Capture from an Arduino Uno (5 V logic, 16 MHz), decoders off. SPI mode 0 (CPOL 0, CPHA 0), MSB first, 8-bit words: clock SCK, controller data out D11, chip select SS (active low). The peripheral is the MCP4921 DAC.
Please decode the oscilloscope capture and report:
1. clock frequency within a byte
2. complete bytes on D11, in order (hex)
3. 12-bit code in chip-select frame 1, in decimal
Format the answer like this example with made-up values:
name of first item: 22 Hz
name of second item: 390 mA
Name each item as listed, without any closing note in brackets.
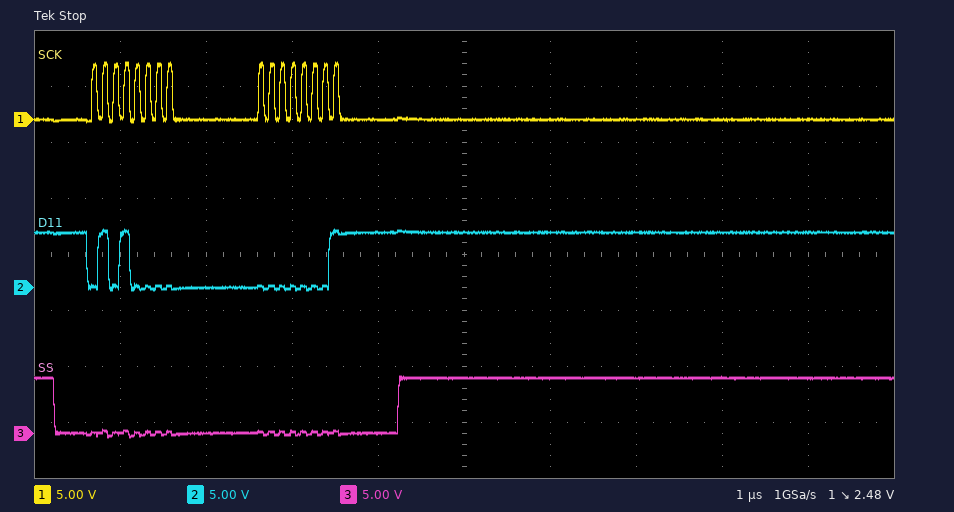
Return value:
clock frequency within a byte: 8 MHz
complete bytes on D11, in order: 0x50 0x01
12-bit code in chip-select frame 1, in decimal: 1
